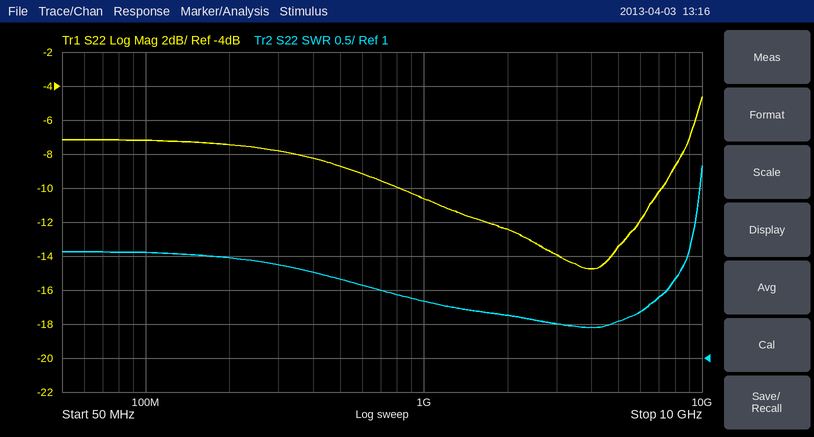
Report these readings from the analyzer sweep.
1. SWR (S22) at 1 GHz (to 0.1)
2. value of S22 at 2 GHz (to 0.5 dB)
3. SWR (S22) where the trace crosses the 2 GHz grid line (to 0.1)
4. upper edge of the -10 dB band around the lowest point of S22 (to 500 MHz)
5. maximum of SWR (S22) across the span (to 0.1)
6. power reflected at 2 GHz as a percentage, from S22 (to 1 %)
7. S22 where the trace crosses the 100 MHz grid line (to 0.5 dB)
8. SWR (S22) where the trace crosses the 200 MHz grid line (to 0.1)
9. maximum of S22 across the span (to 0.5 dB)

1.8
-12.5 dB
1.6
7.0 GHz
3.8
6 %
-7.0 dB
2.5
-4.5 dB
